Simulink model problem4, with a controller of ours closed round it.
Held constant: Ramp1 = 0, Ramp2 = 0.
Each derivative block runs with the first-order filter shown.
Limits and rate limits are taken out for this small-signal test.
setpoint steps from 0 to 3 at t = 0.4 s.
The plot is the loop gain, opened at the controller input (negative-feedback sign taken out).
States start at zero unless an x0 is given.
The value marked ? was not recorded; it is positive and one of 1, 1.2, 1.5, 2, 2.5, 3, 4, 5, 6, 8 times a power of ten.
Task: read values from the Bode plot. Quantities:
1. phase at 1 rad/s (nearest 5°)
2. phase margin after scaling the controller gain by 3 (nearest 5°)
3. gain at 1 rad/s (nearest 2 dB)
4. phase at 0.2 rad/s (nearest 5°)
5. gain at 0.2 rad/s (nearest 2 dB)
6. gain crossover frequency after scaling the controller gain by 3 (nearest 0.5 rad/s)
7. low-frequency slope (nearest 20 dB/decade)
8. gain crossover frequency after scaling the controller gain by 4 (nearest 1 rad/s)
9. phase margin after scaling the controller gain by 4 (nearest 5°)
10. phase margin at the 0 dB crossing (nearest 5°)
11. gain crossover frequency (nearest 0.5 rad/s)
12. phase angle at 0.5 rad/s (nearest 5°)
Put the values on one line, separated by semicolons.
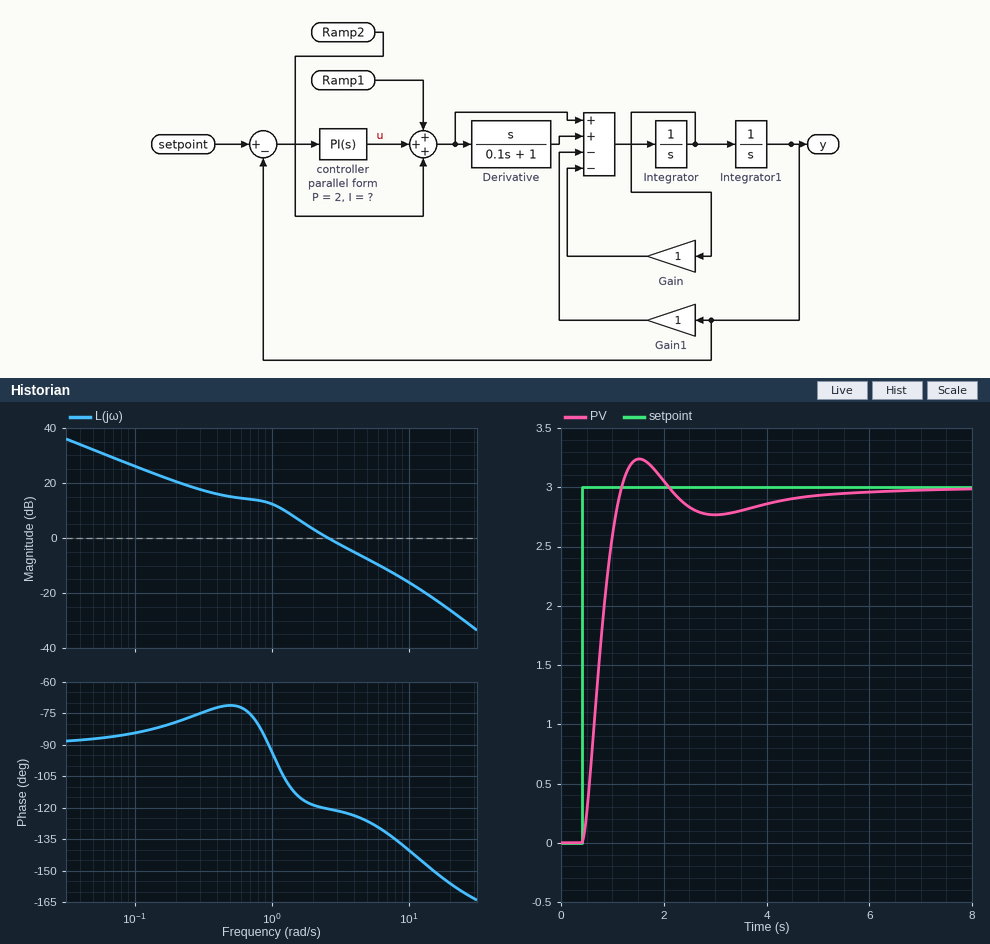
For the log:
-95°; 50°; 12 dB; -80°; 20 dB; 6.0 rad/s; -20 dB/decade; 7 rad/s; 45°; 60°; 2.5 rad/s; -70°
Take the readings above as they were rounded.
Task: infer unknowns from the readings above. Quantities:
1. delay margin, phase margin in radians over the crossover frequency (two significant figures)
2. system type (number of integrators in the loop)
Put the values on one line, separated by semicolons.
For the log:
0.42 s; 1
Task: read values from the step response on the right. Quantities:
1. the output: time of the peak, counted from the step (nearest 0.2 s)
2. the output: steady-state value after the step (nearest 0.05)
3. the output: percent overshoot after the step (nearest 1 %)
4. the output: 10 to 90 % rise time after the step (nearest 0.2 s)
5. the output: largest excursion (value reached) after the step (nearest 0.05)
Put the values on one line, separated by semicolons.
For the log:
1.2 s; 3.00; 8 %; 0.6 s; 3.25
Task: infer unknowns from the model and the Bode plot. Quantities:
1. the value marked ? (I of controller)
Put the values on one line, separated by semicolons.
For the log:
2
